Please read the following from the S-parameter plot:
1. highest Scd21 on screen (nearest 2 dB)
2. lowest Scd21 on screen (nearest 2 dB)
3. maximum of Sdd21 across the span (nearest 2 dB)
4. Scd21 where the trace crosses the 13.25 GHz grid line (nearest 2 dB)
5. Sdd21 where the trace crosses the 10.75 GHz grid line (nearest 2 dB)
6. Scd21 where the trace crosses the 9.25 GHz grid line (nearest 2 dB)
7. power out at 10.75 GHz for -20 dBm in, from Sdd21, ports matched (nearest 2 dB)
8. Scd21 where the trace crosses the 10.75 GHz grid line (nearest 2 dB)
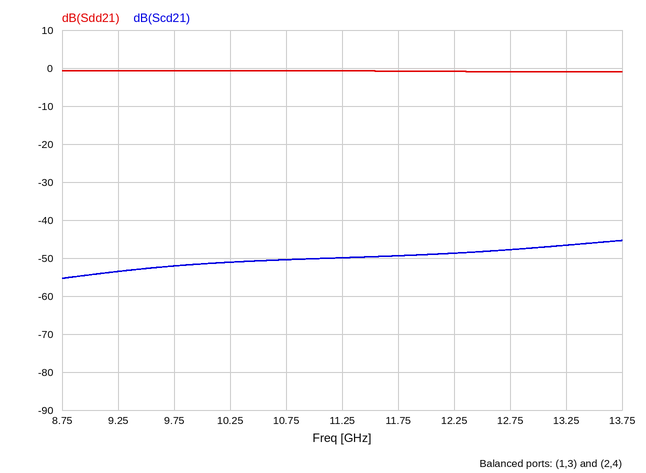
-46 dB
-56 dB
0 dB
-46 dB
0 dB
-54 dB
-20 dBm
-50 dB
